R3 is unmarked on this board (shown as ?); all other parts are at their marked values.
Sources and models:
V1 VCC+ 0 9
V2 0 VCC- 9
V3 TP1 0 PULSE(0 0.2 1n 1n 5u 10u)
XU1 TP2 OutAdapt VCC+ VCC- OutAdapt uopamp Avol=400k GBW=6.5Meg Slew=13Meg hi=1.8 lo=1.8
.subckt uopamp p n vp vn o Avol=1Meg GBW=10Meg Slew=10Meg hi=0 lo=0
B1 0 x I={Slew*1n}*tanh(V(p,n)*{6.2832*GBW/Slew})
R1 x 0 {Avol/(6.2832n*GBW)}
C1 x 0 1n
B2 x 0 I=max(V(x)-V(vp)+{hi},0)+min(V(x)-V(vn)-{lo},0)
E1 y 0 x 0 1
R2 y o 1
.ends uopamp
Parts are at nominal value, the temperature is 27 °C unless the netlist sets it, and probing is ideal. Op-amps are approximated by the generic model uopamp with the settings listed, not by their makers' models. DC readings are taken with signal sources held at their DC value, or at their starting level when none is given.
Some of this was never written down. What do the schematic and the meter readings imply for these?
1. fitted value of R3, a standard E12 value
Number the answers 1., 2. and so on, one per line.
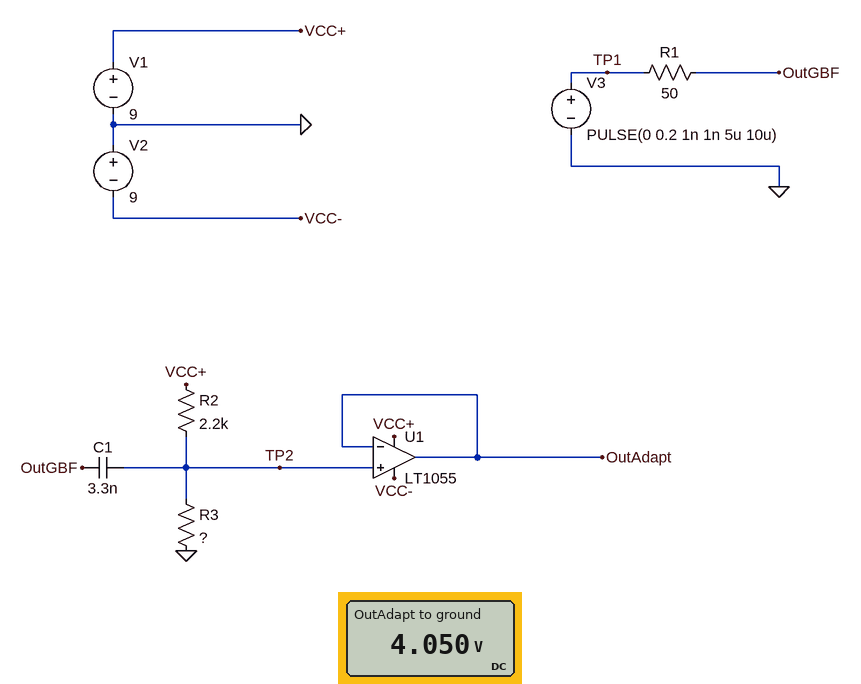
1. 1.8 kΩ
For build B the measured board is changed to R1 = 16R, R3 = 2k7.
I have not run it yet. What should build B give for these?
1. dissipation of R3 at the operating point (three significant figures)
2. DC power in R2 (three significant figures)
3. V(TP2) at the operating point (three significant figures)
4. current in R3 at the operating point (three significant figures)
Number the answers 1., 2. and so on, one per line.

1. 9.11 mW
2. 7.42 mW
3. 4.96 V
4. 1.84 mA
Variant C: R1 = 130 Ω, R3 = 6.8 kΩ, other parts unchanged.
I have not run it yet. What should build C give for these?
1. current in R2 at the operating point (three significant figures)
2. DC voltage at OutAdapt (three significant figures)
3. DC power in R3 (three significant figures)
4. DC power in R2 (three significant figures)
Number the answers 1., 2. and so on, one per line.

1. 1.00 mA
2. 6.80 V
3. 6.80 mW
4. 2.20 mW
